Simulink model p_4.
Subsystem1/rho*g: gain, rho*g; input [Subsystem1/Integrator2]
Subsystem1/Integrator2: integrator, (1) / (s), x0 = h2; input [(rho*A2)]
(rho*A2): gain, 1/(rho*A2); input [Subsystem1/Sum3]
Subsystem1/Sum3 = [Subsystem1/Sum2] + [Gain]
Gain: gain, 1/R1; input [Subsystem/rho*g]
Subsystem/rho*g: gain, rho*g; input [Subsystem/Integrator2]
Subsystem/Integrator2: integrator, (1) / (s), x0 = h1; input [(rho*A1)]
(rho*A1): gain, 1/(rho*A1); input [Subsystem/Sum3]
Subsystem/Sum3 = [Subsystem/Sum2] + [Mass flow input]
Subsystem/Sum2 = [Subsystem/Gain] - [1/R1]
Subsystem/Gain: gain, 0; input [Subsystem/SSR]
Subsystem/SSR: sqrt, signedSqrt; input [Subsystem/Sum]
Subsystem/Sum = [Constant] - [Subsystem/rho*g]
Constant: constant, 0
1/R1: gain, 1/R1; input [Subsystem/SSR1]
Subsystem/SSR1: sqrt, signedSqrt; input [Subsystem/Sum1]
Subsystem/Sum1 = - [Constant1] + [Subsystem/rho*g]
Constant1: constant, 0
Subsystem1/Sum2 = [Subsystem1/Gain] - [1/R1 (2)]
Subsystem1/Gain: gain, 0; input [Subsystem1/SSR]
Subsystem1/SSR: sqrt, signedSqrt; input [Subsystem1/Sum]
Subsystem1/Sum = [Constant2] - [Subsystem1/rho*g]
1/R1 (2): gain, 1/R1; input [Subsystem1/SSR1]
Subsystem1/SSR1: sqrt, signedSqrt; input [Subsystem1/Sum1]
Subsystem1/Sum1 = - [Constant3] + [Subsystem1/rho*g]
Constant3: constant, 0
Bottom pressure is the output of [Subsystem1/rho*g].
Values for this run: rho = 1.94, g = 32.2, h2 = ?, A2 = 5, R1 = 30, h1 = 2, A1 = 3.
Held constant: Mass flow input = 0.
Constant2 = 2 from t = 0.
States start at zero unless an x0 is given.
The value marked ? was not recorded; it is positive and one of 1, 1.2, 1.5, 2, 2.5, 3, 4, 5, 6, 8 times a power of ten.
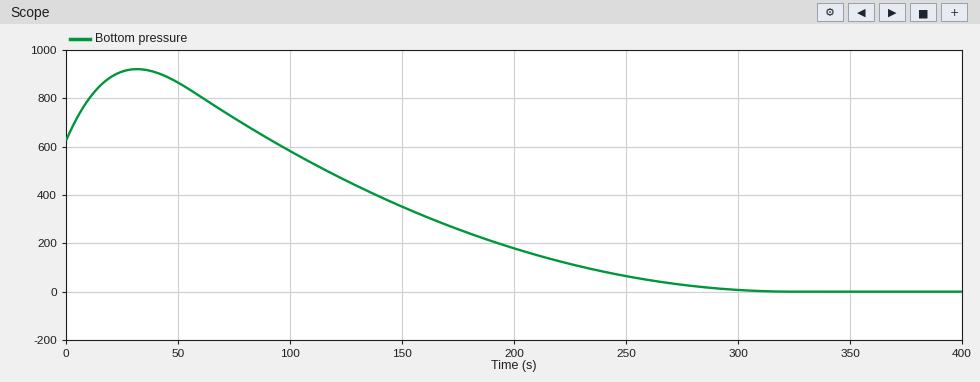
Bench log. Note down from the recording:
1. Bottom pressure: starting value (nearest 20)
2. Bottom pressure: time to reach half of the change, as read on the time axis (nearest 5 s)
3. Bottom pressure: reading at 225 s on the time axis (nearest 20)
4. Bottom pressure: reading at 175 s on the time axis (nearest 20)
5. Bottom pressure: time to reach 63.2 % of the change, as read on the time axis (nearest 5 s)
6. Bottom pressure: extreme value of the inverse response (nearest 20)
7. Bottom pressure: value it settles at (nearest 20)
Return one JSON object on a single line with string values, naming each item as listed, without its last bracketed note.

{"Bottom pressure: starting value": "620", "Bottom pressure: time to reach half of the change, as read on the time axis": "160 s", "Bottom pressure: reading at 225 s on the time axis": "120", "Bottom pressure: reading at 175 s on the time axis": "260", "Bottom pressure: time to reach 63.2 % of the change, as read on the time axis": "185 s", "Bottom pressure: extreme value of the inverse response": "920", "Bottom pressure: value it settles at": "0"}
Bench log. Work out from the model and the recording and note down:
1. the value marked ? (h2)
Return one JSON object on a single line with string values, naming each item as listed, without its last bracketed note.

{"the value marked ?": "10"}
